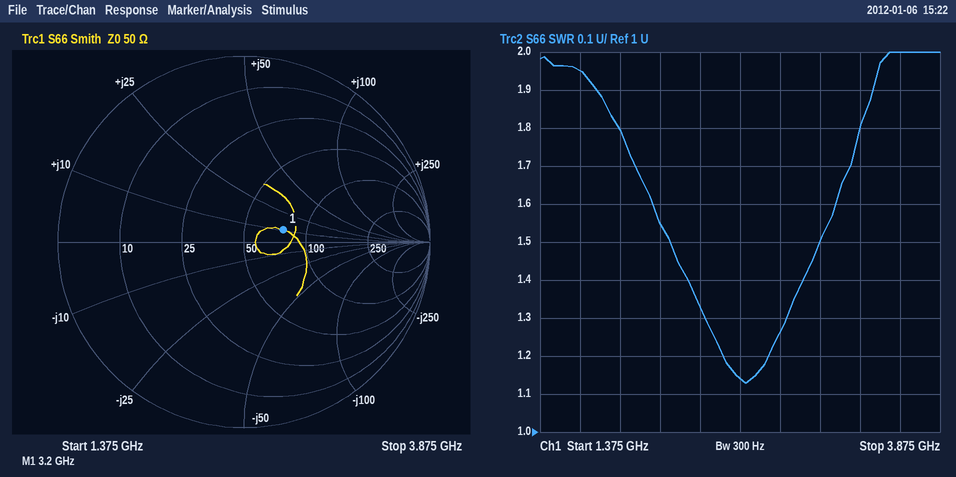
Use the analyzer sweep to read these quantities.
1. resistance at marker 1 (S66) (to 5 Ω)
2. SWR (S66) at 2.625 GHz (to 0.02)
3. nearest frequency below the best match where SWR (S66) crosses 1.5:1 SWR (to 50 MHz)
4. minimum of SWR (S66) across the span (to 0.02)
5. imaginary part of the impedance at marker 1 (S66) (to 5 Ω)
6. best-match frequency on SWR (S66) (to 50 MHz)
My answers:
75 Ω
1.14
2.20 GHz
1.12
+10 Ω
2.65 GHz
